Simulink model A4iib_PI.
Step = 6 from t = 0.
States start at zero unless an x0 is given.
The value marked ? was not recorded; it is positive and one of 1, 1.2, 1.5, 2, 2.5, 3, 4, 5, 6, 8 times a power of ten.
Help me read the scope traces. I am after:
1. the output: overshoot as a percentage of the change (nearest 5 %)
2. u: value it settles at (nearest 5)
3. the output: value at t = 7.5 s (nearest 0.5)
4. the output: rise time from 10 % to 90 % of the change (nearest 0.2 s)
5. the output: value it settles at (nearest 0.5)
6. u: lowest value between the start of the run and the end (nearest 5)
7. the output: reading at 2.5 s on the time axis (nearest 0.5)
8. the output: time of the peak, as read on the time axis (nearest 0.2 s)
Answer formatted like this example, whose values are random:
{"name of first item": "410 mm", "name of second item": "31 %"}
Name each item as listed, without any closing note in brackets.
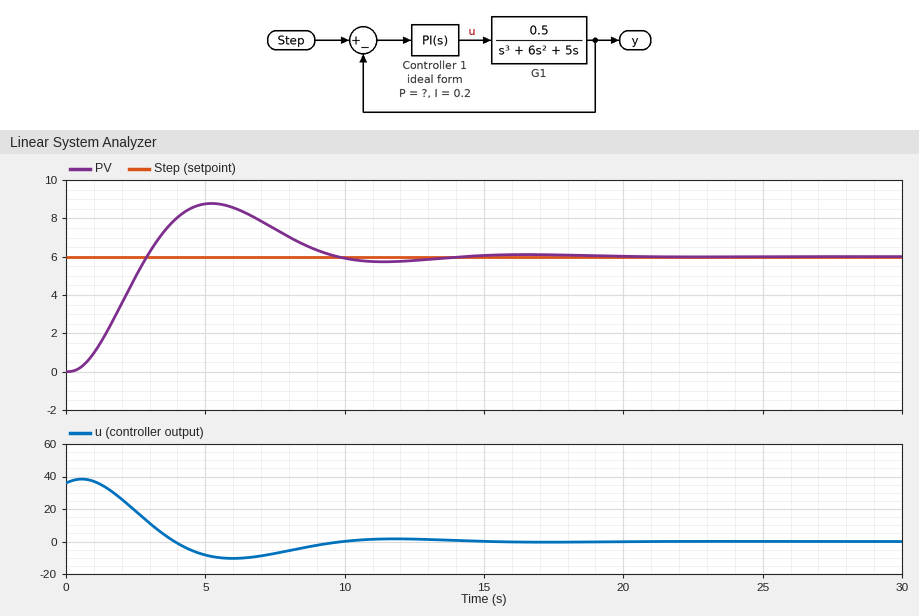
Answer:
{"the output: overshoot as a percentage of the change": "45 %", "u: value it settles at": "0", "the output: value at t = 7.5 s": "7.5", "the output: rise time from 10 % to 90 % of the change": "1.8 s", "the output: value it settles at": "6.0", "u: lowest value between the start of the run and the end": "-10", "the output: reading at 2.5 s on the time axis": "5.0", "the output: time of the peak, as read on the time axis": "5.2 s"}
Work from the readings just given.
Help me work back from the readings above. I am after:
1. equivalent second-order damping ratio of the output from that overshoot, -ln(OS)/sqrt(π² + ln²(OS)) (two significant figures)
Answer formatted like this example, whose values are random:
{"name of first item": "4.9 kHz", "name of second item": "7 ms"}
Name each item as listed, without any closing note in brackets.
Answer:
{"equivalent second-order damping ratio of the output from that overshoot, -ln(OS)/sqrt(π² + ln²(OS))": "0.25"}
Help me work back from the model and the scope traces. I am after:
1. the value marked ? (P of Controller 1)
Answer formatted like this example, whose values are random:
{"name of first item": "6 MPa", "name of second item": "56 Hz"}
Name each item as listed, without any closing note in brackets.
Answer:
{"the value marked ?": "6"}
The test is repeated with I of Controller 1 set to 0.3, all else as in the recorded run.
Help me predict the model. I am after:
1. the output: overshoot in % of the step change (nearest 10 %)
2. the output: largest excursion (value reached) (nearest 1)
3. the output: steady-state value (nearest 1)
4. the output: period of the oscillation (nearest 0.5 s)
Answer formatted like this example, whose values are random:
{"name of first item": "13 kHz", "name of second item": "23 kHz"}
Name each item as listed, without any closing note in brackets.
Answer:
{"the output: overshoot in % of the step change": "60 %", "the output: largest excursion (value reached)": "10", "the output: steady-state value": "6", "the output: period of the oscillation": "11.0 s"}
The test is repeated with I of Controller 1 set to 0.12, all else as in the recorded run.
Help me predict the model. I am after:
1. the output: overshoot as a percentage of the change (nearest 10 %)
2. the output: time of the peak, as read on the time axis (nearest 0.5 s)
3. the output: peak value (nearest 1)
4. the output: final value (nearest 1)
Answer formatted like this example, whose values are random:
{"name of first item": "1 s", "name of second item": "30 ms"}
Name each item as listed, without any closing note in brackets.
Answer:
{"the output: overshoot as a percentage of the change": "30 %", "the output: time of the peak, as read on the time axis": "5.5 s", "the output: peak value": "8", "the output: final value": "6"}
